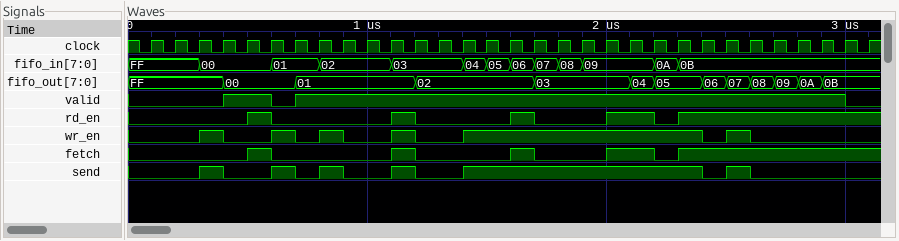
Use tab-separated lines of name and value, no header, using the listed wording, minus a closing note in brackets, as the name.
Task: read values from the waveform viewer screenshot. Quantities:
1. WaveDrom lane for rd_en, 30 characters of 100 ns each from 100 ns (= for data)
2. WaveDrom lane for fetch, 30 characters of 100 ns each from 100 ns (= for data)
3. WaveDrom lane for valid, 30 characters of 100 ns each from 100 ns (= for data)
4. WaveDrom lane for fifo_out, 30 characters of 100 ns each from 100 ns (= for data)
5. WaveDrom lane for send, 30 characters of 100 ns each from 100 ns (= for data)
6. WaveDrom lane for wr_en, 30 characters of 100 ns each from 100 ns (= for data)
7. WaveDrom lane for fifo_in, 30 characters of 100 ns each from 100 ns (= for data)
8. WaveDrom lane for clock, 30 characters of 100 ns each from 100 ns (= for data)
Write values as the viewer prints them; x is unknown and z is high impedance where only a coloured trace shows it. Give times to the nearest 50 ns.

WaveDrom lane for rd_en, 30 characters of 100 ns each from 100 ns	{name: 'rd_en', wave: '0...10....10...10..1.01.......'}
WaveDrom lane for fetch, 30 characters of 100 ns each from 100 ns	{name: 'fetch', wave: '0...10....10...10..1.01.......'}
WaveDrom lane for valid, 30 characters of 100 ns each from 100 ns	{name: 'valid', wave: '0..1.01......................0'}
WaveDrom lane for fifo_out, 30 characters of 100 ns each from 100 ns	{name: 'fifo_out', wave: '=..=..=....=....=...==.======.', data: 'FF 00 01 02 03 04 05 06 07 08 09 0A 0B'}
WaveDrom lane for send, 30 characters of 100 ns each from 100 ns	{name: 'send', wave: '0.10.1010.10.1.........010....'}
WaveDrom lane for wr_en, 30 characters of 100 ns each from 100 ns	{name: 'wr_en', wave: '0.10.1010.10.1.........010....'}
WaveDrom lane for fifo_in, 30 characters of 100 ns each from 100 ns	{name: 'fifo_in', wave: '=.=..=.=..=..======..==.......', data: 'FF 00 01 02 03 04 05 06 07 08 09 0A 0B'}
WaveDrom lane for clock, 30 characters of 100 ns each from 100 ns	{name: 'clock', wave: 'p.............................'}
